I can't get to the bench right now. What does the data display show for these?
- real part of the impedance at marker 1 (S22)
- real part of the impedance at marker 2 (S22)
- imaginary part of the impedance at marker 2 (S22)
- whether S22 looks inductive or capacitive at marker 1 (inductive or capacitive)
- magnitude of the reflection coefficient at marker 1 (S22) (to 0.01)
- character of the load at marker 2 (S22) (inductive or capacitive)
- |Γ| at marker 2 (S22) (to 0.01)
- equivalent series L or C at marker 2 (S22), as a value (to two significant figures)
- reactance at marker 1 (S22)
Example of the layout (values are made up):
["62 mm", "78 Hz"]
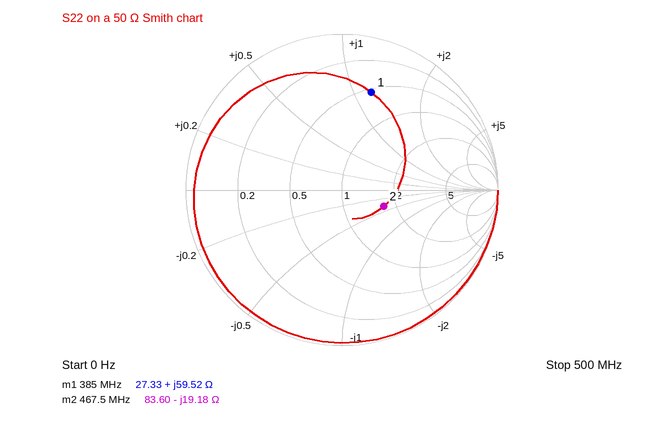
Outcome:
["27.33 Ω", "83.60 Ω", "-19.18 Ω", "inductive", "0.65", "capacitive", "0.29", "18 pF", "+59.52 Ω"]
